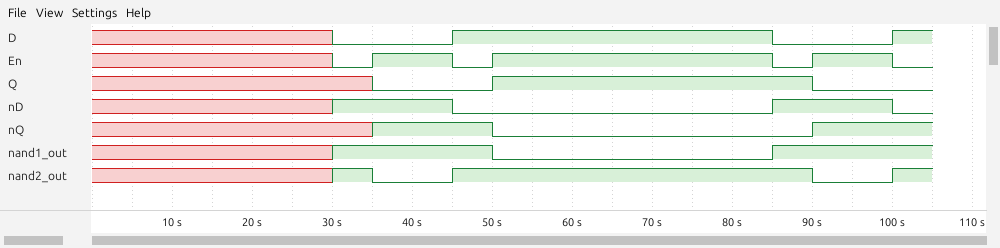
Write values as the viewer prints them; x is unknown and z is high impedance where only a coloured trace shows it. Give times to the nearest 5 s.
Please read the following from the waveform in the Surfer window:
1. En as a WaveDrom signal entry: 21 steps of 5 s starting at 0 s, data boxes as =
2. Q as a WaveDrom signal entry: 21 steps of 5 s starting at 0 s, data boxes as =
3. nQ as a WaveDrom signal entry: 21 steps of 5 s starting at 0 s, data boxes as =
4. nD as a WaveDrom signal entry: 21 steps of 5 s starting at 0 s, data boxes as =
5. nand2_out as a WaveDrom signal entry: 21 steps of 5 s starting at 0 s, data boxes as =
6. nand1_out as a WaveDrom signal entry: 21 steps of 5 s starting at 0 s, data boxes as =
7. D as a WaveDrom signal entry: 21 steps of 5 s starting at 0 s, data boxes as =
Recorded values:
{name: 'En', wave: 'x.....01.01......01.0'}
{name: 'Q', wave: 'x......0..1.......0..'}
{name: 'nQ', wave: 'x......1..0.......1..'}
{name: 'nD', wave: 'x.....1..0.......1..0'}
{name: 'nand2_out', wave: 'x.....10.1........0.1'}
{name: 'nand1_out', wave: 'x.....1...0......1...'}
{name: 'D', wave: 'x.....0..1.......0..1'}
